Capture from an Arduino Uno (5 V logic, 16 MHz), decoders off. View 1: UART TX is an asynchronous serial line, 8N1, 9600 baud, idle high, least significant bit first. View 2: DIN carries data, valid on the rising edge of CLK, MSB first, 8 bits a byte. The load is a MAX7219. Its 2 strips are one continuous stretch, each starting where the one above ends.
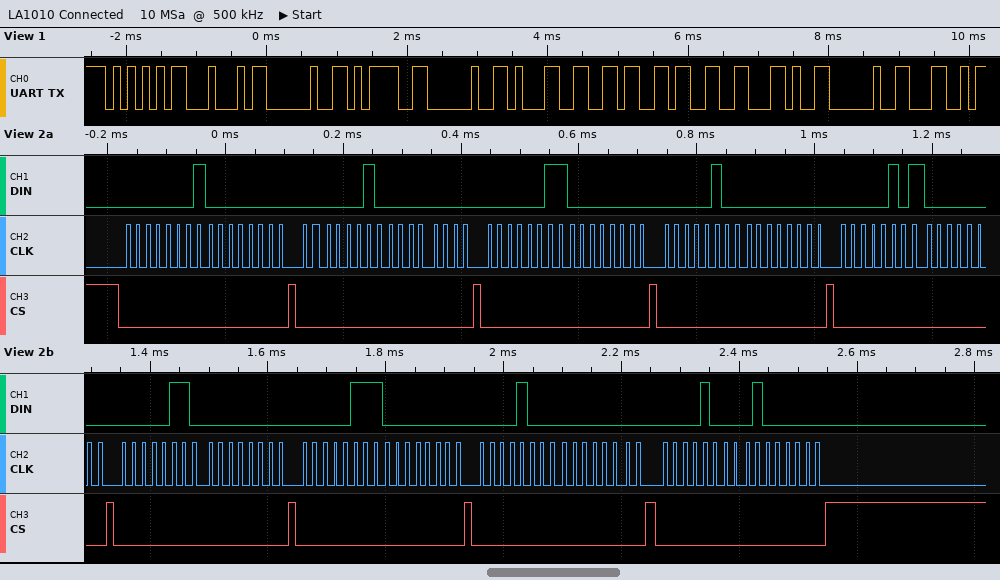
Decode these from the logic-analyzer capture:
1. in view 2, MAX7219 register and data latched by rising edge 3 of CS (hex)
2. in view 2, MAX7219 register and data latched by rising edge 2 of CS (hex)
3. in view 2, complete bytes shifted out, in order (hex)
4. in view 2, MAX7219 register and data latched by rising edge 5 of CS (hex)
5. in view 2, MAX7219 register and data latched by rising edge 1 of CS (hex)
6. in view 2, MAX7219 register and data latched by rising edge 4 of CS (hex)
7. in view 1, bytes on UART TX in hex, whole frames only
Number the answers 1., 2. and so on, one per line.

1. register 0x3, data 0x00
2. register 0x2, data 0x00
3. 01 00 02 00 03 00 04 00 05 00 06 00 07 00 08 00 08 40
4. register 0x5, data 0x00
5. register 0x1, data 0x00
6. register 0x4, data 0x00
7. 55 44 20 3D 20 31 36 33 2C 20 4C
